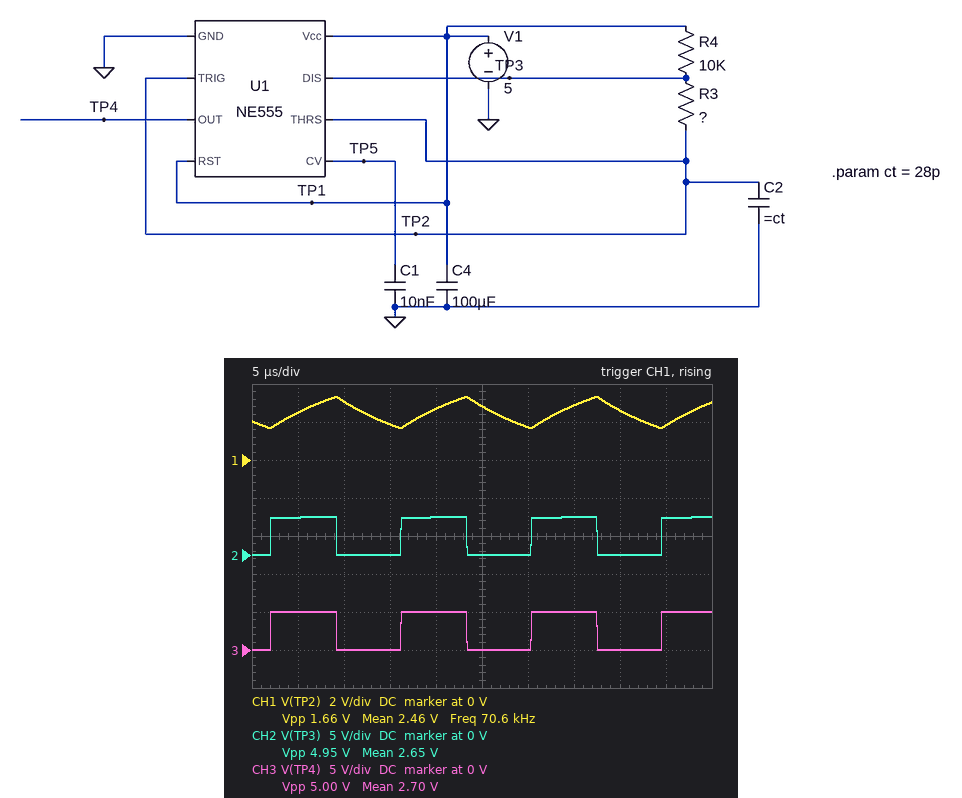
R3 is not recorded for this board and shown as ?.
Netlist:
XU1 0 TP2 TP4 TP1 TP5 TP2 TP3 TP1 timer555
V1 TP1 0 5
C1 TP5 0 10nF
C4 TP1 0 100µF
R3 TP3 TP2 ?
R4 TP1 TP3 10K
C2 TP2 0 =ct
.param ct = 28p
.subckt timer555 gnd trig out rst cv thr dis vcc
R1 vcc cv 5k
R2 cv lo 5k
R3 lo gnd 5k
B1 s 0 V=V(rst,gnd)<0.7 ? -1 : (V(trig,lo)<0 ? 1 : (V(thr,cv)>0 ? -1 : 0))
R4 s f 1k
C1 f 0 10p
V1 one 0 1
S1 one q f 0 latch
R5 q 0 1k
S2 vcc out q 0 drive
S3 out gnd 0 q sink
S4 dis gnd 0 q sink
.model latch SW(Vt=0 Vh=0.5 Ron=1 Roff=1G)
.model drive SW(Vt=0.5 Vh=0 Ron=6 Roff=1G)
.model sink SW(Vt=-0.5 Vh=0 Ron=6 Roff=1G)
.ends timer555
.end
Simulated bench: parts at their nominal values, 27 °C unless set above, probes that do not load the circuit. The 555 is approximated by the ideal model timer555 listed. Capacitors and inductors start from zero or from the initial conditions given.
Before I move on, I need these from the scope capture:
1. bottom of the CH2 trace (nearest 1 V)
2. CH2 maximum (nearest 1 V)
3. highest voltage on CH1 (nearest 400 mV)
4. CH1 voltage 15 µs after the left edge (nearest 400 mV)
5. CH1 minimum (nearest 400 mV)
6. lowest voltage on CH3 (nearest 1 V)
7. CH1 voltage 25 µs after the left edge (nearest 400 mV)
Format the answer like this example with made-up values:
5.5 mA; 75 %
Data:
0 V; 5 V; 3.2 V; 2.0 V; 1.6 V; 0 V; 2.8 V
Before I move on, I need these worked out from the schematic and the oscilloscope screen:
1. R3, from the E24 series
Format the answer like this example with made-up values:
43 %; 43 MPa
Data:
360 kΩ
